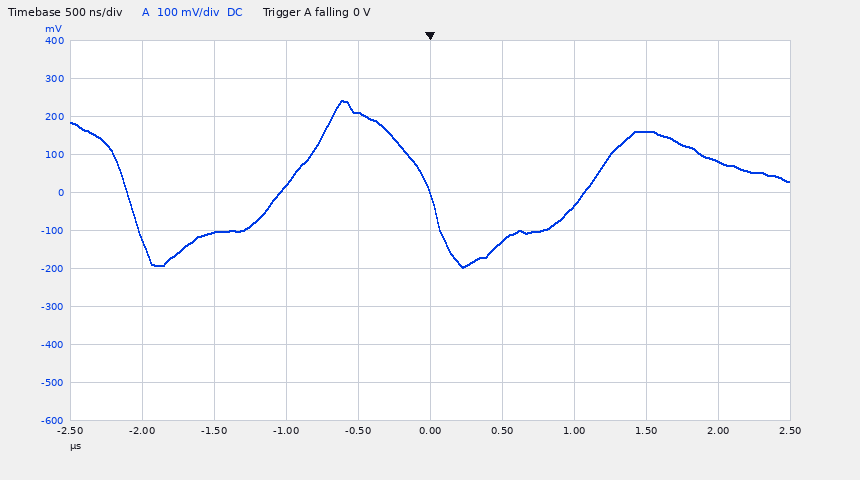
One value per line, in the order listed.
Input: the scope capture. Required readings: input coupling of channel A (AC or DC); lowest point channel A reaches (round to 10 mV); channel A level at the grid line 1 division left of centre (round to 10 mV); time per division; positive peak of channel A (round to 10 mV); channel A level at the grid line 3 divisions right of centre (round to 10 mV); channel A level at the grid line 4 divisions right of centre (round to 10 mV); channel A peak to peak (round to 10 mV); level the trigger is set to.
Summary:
DC
-200 mV
210 mV
500 ns
240 mV
160 mV
80 mV
440 mV
0 V
